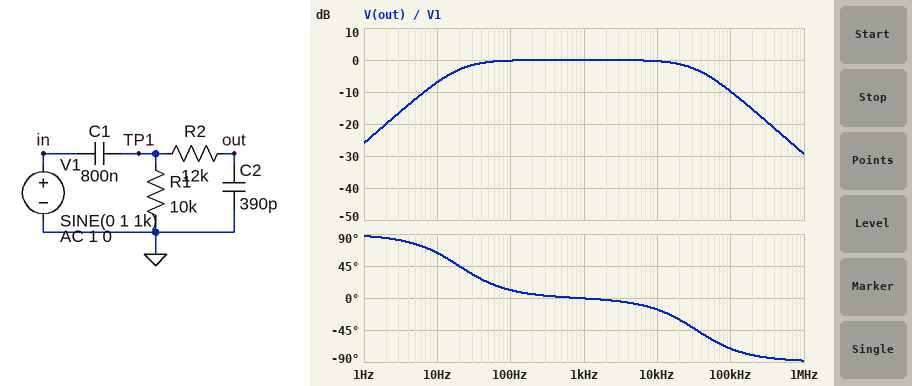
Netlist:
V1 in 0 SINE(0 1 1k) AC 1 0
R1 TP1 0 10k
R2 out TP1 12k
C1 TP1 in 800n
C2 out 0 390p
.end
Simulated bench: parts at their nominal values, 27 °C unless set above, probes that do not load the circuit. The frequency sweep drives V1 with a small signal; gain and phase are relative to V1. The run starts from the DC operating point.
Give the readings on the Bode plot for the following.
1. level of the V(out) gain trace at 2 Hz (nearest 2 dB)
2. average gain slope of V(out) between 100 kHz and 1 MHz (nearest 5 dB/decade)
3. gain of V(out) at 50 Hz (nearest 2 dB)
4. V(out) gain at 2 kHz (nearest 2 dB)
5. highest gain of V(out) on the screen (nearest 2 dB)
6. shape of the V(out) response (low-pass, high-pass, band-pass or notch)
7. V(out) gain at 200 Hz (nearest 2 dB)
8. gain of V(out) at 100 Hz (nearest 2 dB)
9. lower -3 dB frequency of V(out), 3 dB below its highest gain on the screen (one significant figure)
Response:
-20 dB
-20 dB/decade
0 dB
0 dB
0 dB
band-pass
0 dB
0 dB
20 Hz
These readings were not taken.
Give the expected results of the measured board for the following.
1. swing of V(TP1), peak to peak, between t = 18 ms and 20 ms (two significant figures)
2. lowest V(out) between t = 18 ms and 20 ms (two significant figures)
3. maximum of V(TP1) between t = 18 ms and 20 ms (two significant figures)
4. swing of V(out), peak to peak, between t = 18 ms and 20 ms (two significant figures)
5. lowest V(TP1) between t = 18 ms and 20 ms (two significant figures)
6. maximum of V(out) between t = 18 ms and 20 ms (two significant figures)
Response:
2.0 V
-1.0 V
1.0 V
2.0 V
-1.0 V
1.0 V
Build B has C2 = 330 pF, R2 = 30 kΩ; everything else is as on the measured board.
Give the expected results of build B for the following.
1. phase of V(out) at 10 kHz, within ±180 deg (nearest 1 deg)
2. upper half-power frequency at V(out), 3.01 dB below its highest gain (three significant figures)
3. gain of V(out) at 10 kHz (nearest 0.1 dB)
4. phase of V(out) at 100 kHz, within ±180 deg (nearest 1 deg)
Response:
-32 deg
16.1 kHz
-1.4 dB
-81 deg
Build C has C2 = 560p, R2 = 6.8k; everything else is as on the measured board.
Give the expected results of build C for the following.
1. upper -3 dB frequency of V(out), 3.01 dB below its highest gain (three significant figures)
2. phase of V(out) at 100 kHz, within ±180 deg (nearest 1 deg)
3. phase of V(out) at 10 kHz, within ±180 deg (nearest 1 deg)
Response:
41.9 kHz
-67 deg
-13 deg
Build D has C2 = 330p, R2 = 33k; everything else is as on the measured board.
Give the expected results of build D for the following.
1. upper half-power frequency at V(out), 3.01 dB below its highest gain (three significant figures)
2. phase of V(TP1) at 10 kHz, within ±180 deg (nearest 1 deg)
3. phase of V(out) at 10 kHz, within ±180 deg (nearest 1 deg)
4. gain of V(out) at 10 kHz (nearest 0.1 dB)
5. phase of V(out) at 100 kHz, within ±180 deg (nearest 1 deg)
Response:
14.7 kHz
0 deg
-34 deg
-1.7 dB
-82 deg
